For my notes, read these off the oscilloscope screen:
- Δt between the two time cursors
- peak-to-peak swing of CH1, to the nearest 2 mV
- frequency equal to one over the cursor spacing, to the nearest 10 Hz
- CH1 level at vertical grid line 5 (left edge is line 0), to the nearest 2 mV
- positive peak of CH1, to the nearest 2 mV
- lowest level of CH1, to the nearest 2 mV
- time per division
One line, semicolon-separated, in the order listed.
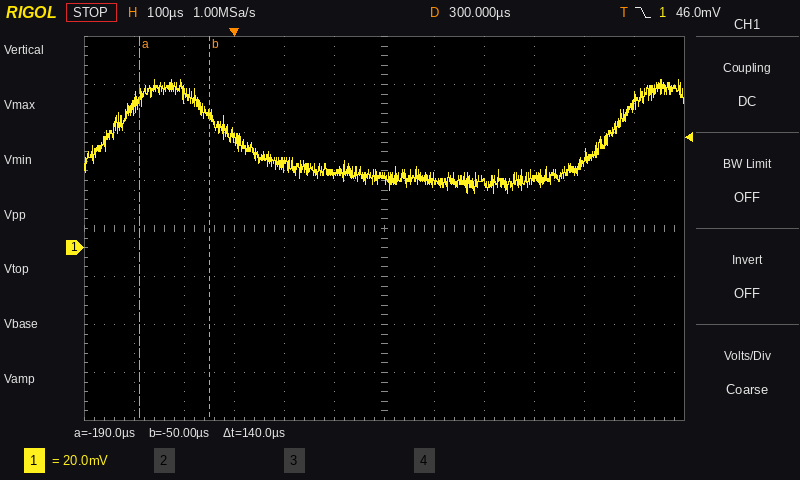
140 µs; 48 mV; 7.14 kHz; 30 mV; 70 mV; 22 mV; 100 µs
